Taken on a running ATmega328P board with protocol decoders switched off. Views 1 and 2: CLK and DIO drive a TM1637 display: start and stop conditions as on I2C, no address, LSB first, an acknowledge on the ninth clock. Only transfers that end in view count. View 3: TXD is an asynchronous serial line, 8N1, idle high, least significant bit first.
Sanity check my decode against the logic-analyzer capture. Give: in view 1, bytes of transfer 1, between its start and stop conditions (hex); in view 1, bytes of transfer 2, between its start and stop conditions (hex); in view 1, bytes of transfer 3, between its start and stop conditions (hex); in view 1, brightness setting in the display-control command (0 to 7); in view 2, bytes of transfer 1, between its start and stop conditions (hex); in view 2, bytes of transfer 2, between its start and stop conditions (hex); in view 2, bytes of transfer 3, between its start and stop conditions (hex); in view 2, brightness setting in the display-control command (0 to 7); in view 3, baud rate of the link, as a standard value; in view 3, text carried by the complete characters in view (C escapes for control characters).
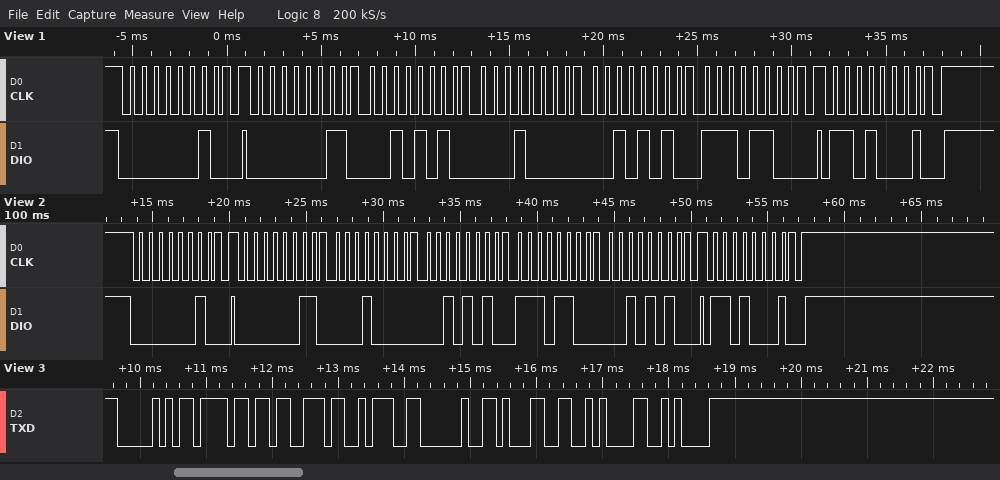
40
C0 54 08 54 37
8B
3
40
C0 08 54 37 54
8B
3
9600 baud
"Pos: 1\n\n"
